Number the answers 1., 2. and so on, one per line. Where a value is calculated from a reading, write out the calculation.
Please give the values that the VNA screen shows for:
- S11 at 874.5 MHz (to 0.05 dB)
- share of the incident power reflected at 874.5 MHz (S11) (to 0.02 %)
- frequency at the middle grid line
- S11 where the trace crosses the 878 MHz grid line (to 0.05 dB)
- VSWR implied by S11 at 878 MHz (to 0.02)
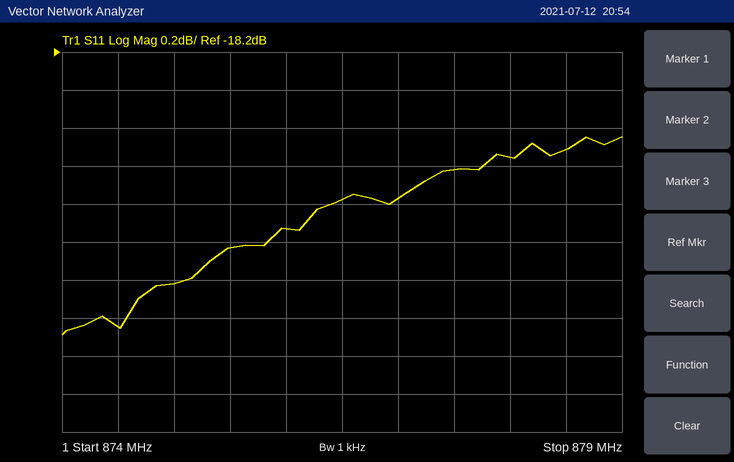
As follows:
1. -19.65 dB
2. 10^(-19.65/10) ≈ 1.08 %
3. 876.5 MHz
4. -18.75 dB
5. |Γ| = 10^(-18.75/20) = 0.1155; VSWR = (1 + 0.1155)/(1 − 0.1155) ≈ 1.26
